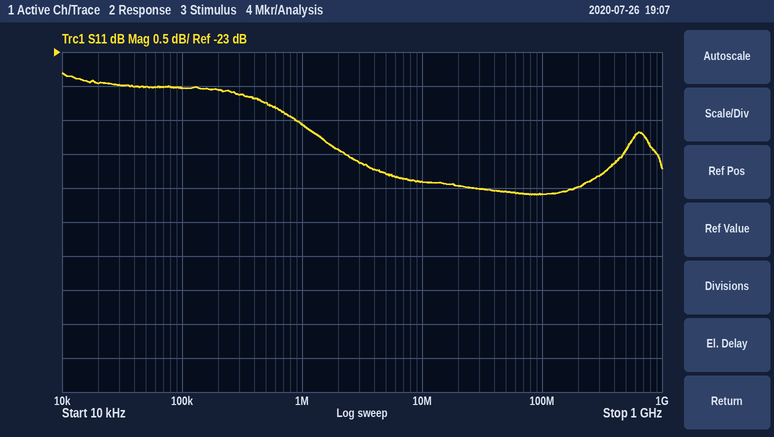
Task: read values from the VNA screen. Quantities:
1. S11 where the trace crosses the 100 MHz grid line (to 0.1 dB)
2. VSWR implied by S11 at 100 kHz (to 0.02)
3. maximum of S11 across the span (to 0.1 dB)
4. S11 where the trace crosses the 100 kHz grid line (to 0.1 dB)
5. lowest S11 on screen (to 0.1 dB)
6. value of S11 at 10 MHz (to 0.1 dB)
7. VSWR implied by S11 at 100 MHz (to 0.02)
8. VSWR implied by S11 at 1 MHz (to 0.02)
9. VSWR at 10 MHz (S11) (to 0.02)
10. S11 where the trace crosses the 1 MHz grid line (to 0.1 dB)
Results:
-25.1 dB
1.14
-23.3 dB
-23.5 dB
-25.1 dB
-24.9 dB
1.12
1.14
1.12
-24.1 dB
